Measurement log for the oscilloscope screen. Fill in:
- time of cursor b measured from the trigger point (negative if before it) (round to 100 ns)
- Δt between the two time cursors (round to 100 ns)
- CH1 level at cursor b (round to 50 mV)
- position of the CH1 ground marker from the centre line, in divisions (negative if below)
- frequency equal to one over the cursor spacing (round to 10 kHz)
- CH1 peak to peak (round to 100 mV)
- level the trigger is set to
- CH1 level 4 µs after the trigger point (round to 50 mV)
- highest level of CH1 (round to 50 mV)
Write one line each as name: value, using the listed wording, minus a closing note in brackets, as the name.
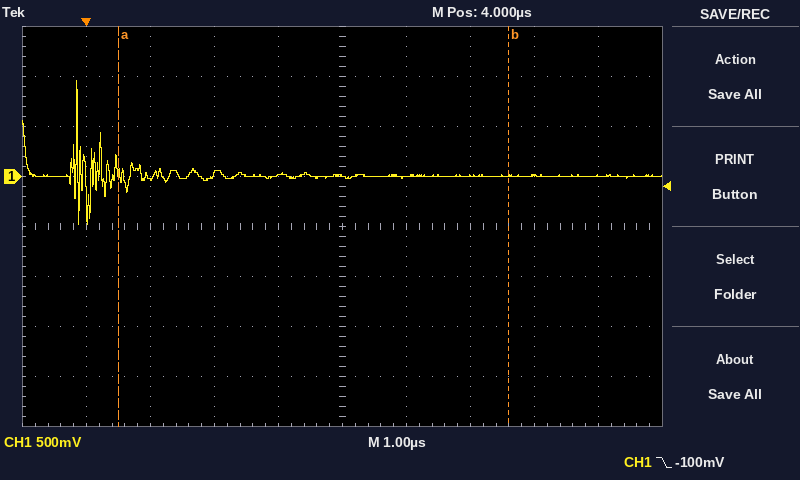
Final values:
time of cursor b measured from the trigger point (negative if before it): +6.6 µs
Δt between the two time cursors: 6.1 µs
CH1 level at cursor b: 0 mV
position of the CH1 ground marker from the centre line, in divisions: +1.0 div
frequency equal to one over the cursor spacing: 160 kHz
CH1 peak to peak: 1.40 V
level the trigger is set to: -100 mV
CH1 level 4 µs after the trigger point: 0 mV
highest level of CH1: 950 mV
